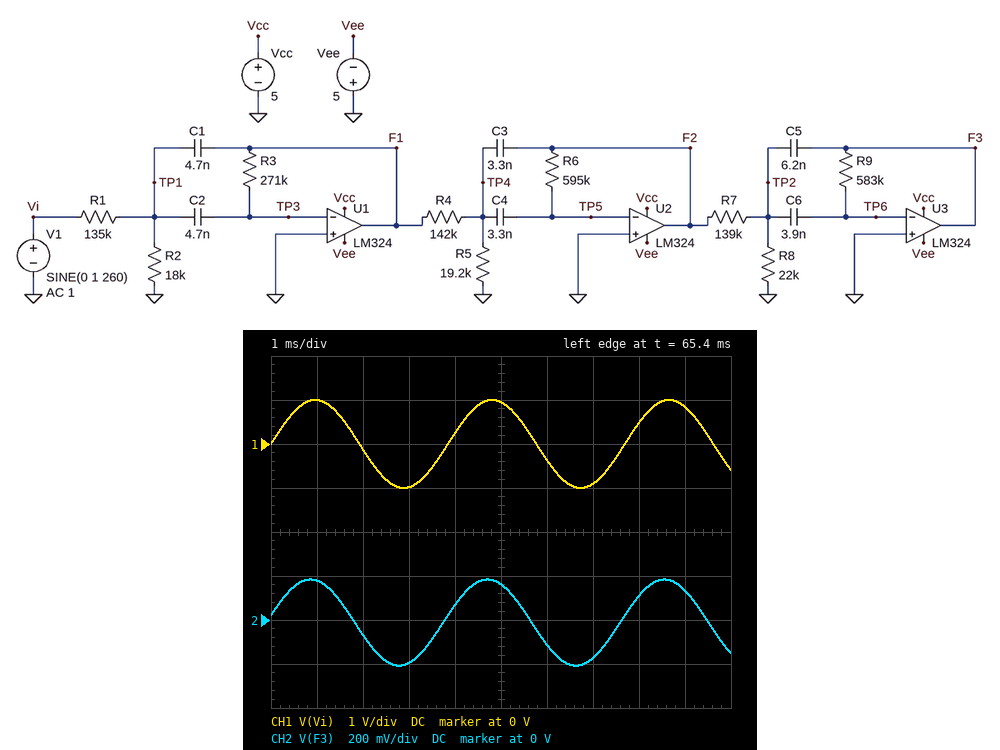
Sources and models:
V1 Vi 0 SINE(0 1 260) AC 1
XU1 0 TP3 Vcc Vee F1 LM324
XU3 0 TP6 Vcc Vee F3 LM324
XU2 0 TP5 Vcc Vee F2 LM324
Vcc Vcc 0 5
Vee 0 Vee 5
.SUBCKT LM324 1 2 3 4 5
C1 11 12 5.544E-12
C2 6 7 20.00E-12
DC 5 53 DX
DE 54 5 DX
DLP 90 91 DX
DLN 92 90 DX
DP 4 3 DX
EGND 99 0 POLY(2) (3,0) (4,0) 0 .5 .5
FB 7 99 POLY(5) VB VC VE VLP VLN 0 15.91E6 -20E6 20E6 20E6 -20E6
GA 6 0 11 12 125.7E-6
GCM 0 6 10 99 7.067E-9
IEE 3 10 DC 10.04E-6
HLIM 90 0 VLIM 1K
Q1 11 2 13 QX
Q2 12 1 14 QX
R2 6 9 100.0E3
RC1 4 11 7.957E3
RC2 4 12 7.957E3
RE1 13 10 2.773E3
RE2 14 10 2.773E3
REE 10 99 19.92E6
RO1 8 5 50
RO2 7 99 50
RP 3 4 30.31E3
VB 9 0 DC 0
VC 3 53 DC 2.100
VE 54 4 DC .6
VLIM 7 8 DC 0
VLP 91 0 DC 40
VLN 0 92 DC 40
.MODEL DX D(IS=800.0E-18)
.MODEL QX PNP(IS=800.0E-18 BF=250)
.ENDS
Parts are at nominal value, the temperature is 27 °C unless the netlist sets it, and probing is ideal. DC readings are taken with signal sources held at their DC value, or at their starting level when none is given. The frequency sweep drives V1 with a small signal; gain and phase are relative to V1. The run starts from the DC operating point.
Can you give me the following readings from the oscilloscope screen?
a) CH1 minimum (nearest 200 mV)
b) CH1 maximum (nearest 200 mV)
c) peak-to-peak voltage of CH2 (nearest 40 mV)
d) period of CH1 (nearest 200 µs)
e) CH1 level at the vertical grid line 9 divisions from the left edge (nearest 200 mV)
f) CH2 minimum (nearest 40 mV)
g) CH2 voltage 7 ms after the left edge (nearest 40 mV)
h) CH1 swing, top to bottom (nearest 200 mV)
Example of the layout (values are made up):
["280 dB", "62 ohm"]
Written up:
["-1.0 V", "1.0 V", "400 mV", "3.8 ms", "800 mV", "-200 mV", "-160 mV", "2.0 V"]
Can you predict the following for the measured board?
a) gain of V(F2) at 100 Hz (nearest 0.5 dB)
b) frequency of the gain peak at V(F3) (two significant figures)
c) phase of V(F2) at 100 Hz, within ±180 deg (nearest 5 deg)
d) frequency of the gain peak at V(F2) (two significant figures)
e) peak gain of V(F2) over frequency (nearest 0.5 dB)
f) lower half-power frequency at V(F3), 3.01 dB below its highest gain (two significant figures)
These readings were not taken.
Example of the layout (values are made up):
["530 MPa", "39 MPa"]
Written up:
["-36.5 dB", "470 Hz", "170 deg", "490 Hz", "6.0 dB", "390 Hz"]
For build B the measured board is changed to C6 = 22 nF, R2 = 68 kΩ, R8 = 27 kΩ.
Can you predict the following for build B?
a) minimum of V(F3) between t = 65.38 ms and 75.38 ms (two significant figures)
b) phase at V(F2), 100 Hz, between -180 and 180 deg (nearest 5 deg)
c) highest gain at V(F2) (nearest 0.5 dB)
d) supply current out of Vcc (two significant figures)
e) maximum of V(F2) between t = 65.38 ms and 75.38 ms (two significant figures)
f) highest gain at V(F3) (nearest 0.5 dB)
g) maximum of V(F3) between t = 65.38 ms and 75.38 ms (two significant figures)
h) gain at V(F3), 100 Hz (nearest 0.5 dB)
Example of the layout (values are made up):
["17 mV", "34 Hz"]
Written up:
["-430 mV", "160 deg", "3.0 dB", "1.0 mA", "480 mV", "-4.0 dB", "410 mV", "-18.5 dB"]
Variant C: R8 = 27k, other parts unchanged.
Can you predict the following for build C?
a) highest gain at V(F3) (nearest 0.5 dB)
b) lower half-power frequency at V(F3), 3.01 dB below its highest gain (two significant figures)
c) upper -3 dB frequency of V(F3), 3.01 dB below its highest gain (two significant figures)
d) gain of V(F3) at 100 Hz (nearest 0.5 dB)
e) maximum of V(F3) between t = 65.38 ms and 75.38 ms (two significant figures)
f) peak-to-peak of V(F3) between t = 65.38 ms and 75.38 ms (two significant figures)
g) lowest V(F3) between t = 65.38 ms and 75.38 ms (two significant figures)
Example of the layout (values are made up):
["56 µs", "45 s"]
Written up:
["1.0 dB", "400 Hz", "540 Hz", "-48.0 dB", "230 mV", "490 mV", "-260 mV"]
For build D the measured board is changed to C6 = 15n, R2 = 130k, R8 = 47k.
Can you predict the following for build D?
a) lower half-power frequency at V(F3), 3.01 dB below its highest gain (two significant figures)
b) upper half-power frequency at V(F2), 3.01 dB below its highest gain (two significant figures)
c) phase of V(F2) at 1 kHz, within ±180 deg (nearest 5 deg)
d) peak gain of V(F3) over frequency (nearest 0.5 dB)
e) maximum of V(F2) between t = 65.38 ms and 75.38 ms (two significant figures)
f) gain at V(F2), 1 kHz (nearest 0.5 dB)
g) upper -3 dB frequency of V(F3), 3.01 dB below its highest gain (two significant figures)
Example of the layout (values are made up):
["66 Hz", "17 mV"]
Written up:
["180 Hz", "540 Hz", "-155 deg", "-5.5 dB", "510 mV", "-19.0 dB", "520 Hz"]
